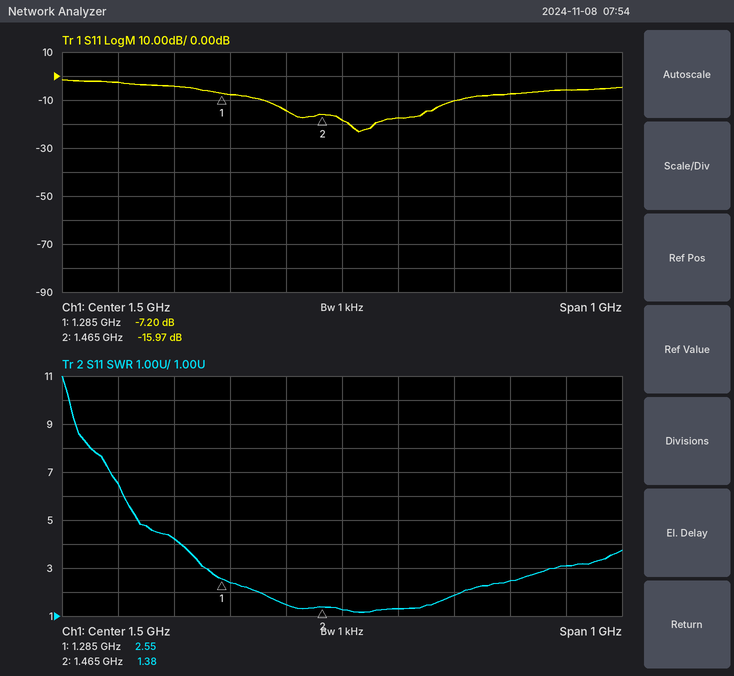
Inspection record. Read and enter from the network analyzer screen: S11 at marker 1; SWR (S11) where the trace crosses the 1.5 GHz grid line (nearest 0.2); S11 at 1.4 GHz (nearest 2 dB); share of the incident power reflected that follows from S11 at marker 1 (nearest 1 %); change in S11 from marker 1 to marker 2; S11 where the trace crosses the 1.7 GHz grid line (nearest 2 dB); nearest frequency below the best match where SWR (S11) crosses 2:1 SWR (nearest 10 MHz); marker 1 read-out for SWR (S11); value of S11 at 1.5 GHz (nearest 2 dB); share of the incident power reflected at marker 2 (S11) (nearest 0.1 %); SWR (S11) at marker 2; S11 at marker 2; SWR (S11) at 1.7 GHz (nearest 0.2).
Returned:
-7.20 dB
1.2
-14 dB
19 %
-8.77 dB
-10 dB
1.35 GHz
2.55
-18 dB
2.5 %
1.38
-15.97 dB
1.8
